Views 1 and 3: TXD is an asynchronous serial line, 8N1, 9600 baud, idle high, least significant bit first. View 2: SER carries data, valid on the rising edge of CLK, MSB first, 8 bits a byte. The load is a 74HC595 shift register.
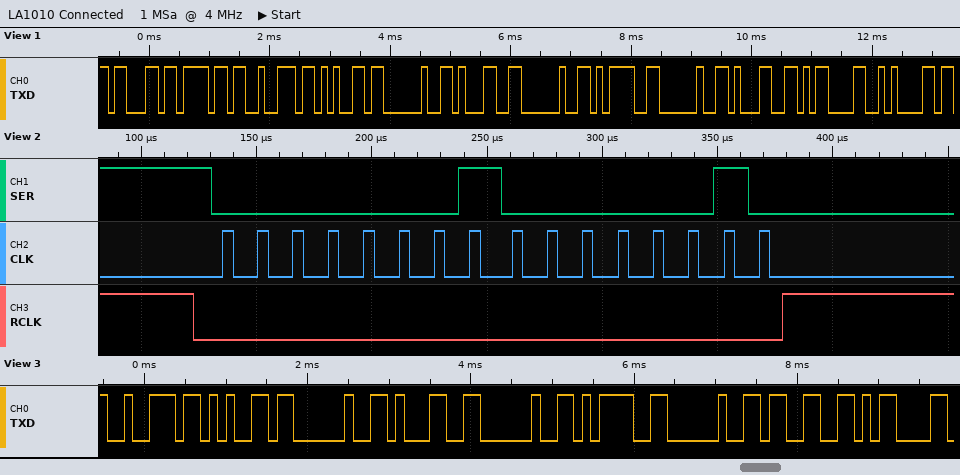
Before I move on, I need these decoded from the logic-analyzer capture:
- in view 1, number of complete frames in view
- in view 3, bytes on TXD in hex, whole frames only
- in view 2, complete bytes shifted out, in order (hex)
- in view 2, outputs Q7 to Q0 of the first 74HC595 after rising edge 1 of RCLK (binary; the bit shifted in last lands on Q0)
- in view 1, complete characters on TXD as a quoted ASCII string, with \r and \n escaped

12
72 65 20 31 20 3D 20 33 0D
0x01 0x02
00000010
"core 1 = 1\r\n"
